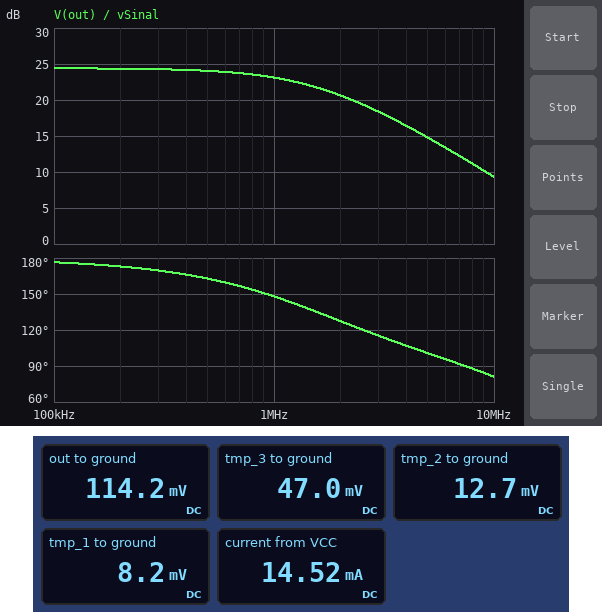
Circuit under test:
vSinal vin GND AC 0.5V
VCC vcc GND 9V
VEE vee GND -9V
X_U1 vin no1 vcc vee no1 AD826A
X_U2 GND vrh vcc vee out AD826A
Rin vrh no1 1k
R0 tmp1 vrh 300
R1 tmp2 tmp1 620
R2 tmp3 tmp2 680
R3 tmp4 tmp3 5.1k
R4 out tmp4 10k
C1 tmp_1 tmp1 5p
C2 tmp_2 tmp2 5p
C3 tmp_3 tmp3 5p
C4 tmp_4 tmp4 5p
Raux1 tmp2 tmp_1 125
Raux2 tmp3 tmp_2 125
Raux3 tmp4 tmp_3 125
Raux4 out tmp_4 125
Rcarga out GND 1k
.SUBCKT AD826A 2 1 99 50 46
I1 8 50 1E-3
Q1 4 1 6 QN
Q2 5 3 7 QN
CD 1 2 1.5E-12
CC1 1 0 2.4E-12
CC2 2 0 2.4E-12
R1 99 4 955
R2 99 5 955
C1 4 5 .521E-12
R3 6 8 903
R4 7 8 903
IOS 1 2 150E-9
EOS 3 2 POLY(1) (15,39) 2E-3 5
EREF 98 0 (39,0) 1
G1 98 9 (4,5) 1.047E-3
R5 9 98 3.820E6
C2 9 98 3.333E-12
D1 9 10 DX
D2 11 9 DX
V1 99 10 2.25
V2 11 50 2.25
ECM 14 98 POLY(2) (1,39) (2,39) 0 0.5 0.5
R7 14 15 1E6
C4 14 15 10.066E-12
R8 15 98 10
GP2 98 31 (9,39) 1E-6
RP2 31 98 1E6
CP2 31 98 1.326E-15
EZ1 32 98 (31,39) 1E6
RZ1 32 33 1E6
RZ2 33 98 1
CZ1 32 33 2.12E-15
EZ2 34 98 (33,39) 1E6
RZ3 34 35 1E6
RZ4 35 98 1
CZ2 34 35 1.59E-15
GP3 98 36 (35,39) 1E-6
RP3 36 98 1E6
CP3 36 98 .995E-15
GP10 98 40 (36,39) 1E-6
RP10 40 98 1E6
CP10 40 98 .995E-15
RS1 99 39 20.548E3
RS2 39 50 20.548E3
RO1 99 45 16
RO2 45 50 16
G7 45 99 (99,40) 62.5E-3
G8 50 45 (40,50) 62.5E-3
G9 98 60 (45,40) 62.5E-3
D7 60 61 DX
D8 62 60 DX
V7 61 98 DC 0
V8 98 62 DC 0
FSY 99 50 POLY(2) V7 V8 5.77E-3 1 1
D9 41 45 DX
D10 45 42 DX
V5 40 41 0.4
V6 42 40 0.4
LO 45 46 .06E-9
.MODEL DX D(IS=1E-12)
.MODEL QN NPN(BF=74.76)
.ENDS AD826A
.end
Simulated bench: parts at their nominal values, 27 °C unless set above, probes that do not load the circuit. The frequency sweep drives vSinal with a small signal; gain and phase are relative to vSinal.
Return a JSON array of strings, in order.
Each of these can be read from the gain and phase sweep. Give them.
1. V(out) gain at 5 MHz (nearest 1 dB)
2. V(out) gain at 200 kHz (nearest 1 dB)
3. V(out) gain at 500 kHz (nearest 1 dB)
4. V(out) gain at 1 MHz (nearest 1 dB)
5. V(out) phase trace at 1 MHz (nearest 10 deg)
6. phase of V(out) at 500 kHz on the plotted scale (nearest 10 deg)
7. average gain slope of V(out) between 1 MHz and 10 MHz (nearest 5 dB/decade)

["15 dB", "24 dB", "24 dB", "23 dB", "150 deg", "160 deg", "-15 dB/decade"]
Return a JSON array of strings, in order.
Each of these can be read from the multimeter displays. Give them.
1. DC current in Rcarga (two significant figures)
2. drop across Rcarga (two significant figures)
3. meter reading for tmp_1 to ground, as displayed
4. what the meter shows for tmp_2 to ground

["110 µA", "110 mV", "8.2 mV", "12.7 mV"]
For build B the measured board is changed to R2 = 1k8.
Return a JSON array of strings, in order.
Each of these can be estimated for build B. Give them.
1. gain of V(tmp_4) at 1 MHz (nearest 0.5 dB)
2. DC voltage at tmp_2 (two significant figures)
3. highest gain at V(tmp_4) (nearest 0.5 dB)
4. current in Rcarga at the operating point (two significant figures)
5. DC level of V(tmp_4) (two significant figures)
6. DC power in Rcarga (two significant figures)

["23.5 dB", "20 mV", "25.0 dB", "120 µA", "120 mV", "15 µW"]
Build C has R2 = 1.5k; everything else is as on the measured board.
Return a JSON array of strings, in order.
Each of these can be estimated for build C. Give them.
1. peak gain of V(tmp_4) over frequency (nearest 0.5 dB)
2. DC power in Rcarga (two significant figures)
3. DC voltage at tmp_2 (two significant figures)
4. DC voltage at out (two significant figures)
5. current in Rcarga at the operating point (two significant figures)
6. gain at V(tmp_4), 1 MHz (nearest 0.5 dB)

["25.0 dB", "14 µW", "18 mV", "120 mV", "120 µA", "23.5 dB"]
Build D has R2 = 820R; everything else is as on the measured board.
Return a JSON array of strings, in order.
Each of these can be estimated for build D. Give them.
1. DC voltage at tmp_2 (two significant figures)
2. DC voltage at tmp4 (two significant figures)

["14 mV", "48 mV"]
